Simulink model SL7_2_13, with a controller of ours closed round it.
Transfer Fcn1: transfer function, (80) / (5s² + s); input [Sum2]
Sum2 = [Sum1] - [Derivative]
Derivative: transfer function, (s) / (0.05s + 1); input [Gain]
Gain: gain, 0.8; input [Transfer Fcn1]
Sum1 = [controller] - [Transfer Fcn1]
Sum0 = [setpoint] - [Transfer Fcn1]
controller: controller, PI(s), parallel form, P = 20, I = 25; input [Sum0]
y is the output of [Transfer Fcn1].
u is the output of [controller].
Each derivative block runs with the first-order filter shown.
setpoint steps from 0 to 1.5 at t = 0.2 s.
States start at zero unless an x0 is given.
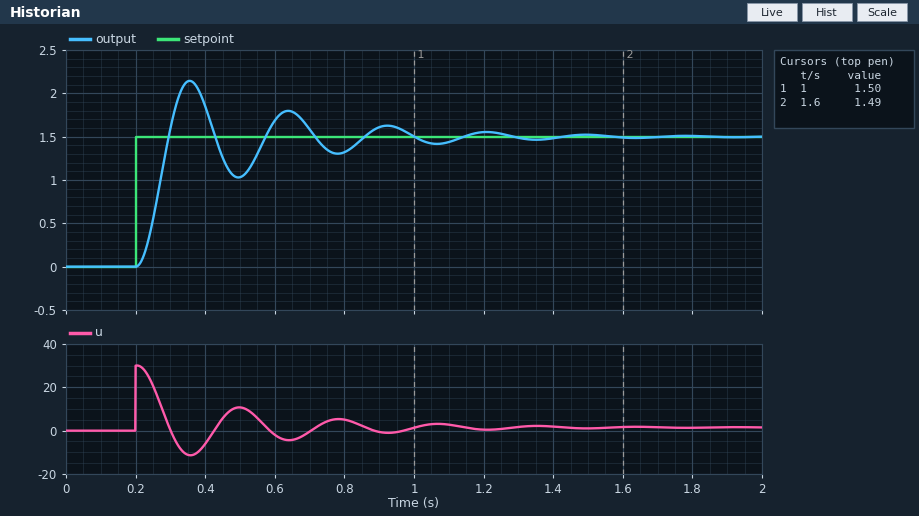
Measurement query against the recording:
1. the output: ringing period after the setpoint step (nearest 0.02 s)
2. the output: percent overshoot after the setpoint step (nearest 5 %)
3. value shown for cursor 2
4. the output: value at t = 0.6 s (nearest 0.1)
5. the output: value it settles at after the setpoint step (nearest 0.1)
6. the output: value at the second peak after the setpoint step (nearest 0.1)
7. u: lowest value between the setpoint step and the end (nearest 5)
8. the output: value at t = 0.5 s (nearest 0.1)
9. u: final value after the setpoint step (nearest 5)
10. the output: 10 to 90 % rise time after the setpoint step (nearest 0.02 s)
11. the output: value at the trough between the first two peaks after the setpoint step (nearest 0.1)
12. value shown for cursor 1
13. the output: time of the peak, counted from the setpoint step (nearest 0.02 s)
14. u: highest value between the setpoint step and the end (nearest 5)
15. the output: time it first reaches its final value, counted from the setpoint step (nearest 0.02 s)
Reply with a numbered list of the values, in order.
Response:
1. 0.28 s
2. 45 %
3. 1.49
4. 1.7
5. 1.5
6. 1.8
7. -10
8. 1.0
9. 0
10. 0.06 s
11. 1.0
12. 1.50
13. 0.16 s
14. 30
15. 0.10 s
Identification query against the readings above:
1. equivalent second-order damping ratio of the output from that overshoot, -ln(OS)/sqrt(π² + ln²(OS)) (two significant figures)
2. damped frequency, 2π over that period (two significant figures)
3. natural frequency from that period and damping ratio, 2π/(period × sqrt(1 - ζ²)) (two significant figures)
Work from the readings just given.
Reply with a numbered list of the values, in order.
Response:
1. 0.25
2. 22 rad/s
3. 23 rad/s
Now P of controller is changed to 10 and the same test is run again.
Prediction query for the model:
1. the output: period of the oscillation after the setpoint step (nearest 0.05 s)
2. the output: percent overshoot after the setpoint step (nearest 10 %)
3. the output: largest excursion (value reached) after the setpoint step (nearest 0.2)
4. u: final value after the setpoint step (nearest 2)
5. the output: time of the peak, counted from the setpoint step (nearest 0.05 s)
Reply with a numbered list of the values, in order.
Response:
1. 0.35 s
2. 30 %
3. 2.0
4. 2
5. 0.20 s
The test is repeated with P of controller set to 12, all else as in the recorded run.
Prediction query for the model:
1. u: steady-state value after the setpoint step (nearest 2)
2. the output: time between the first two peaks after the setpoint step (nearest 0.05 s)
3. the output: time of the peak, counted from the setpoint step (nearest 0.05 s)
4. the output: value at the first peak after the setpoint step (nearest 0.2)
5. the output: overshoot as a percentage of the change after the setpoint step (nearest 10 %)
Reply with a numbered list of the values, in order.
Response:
1. 2
2. 0.35 s
3. 0.20 s
4. 2.0
5. 30 %
